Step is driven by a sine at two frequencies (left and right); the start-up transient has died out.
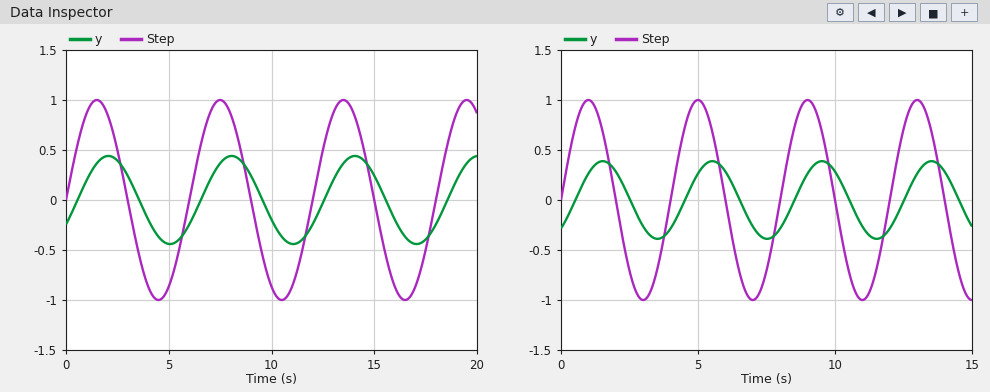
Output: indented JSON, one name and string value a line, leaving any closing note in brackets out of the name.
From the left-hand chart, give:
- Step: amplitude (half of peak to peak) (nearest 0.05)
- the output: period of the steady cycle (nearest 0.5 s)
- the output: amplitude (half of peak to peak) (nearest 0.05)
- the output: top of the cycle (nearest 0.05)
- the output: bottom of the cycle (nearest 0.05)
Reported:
{
  "Step: amplitude (half of peak to peak)": "1.00",
  "the output: period of the steady cycle": "6.0 s",
  "the output: amplitude (half of peak to peak)": "0.45",
  "the output: top of the cycle": "0.45",
  "the output: bottom of the cycle": "-0.45"
}
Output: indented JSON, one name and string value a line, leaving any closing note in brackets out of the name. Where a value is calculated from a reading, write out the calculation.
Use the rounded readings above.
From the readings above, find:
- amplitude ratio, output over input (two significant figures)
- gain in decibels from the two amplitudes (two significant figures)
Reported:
{
  "amplitude ratio, output over input": "0.45 / 1 = 0.45",
  "gain in decibels from the two amplitudes": "20 log10(0.45 / 1) = -6.9 dB"
}
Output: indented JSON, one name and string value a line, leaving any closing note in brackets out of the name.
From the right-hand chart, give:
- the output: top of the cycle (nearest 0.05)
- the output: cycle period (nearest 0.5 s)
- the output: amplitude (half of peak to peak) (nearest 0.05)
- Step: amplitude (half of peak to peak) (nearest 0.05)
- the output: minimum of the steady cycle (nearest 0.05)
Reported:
{
  "the output: top of the cycle": "0.40",
  "the output: cycle period": "4.0 s",
  "the output: amplitude (half of peak to peak)": "0.40",
  "Step: amplitude (half of peak to peak)": "1.00",
  "the output: minimum of the steady cycle": "-0.40"
}
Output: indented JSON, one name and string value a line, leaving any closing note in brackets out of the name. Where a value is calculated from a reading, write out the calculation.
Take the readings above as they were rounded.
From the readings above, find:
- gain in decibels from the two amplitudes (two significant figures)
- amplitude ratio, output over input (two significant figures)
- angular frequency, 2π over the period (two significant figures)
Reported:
{
  "gain in decibels from the two amplitudes": "20 log10(0.4 / 1) = -8.0 dB",
  "amplitude ratio, output over input": "0.4 / 1 = 0.40",
  "angular frequency, 2π over the period": "2π / 4 = 1.6 rad/s"
}
